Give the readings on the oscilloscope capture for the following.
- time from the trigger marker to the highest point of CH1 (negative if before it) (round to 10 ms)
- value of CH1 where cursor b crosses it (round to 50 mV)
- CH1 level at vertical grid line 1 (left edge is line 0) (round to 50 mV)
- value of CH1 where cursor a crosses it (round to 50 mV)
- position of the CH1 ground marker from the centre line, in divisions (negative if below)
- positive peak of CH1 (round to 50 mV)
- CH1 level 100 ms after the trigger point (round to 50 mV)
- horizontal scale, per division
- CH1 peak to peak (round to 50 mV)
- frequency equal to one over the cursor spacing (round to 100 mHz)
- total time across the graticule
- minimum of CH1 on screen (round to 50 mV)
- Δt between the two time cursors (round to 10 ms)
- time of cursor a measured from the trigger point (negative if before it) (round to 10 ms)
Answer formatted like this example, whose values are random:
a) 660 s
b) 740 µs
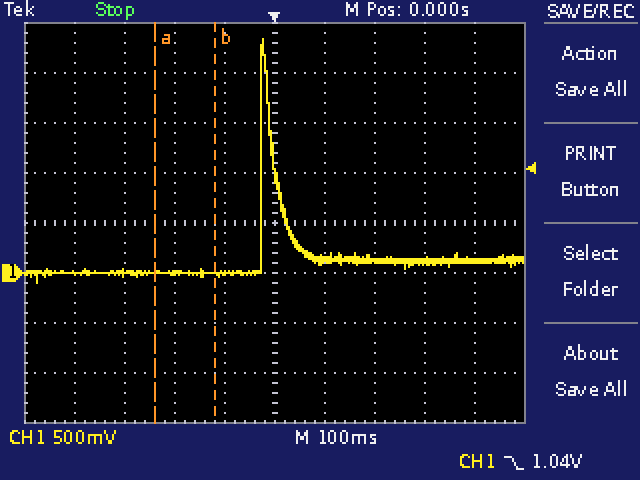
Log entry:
a) -20 ms
b) 0 mV
c) 0 mV
d) 0 mV
e) -1.0 div
f) 2.35 V
g) 150 mV
h) 100 ms
i) 2.45 V
j) 8.3 Hz
k) 1 s
l) -100 mV
m) 120 ms
n) -240 ms
